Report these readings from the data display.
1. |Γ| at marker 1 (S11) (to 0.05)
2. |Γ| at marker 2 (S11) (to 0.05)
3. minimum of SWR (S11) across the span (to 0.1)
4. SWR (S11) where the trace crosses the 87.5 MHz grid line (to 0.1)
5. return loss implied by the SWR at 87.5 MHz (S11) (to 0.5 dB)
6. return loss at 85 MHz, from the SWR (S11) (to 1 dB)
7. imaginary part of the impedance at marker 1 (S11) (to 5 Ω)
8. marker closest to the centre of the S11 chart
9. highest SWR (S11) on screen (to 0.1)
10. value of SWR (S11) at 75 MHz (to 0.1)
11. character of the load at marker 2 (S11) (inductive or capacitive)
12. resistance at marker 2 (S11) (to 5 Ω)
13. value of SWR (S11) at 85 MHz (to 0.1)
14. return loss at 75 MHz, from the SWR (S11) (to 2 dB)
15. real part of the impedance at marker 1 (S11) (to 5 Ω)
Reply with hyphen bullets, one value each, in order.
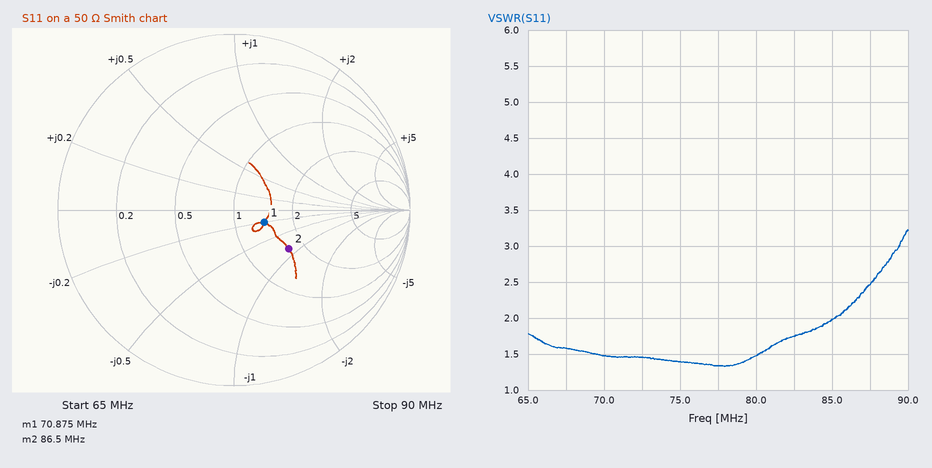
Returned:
- 0.20
- 0.40
- 1.3
- 2.5
- 7.5 dB
- 10 dB
- -10 Ω
- marker 1
- 3.2
- 1.4
- capacitive
- 80 Ω
- 2.0
- 16 dB
- 70 Ω
